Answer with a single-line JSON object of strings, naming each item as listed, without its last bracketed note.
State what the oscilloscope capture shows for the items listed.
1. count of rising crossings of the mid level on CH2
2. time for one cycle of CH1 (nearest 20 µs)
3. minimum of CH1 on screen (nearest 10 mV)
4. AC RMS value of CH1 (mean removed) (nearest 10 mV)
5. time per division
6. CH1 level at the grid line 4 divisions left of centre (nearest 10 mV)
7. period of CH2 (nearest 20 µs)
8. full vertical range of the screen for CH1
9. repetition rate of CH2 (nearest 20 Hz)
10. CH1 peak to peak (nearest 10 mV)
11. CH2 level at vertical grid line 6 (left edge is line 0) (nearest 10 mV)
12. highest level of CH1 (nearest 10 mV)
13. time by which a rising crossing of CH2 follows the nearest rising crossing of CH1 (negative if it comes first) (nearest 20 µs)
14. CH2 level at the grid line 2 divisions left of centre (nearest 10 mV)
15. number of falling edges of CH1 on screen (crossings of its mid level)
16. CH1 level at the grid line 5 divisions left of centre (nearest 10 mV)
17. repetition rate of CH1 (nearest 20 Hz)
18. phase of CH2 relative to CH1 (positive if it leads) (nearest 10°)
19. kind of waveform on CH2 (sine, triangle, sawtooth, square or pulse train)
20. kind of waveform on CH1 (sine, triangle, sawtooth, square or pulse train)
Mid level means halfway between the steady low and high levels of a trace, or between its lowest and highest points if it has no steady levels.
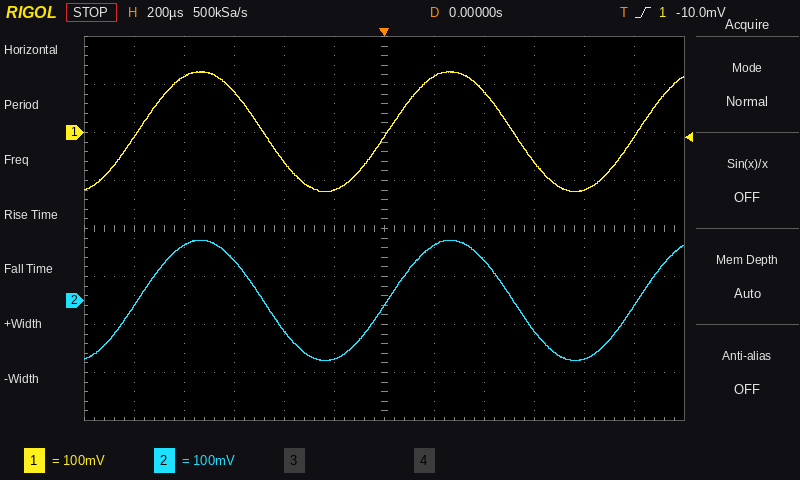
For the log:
{"count of rising crossings of the mid level on CH2": "3", "time for one cycle of CH1": "1.00 ms", "minimum of CH1 on screen": "-120 mV", "AC RMS value of CH1 (mean removed)": "90 mV", "time per division": "200 µs", "CH1 level at the grid line 4 divisions left of centre": "120 mV", "period of CH2": "1.00 ms", "full vertical range of the screen for CH1": "800 mV", "repetition rate of CH2": "1.00 kHz", "CH1 peak to peak": "250 mV", "CH2 level at vertical grid line 6 (left edge is line 0)": "-10 mV", "highest level of CH1": "130 mV", "time by which a rising crossing of CH2 follows the nearest rising crossing of CH1 (negative if it comes first)": "0 µs", "CH2 level at the grid line 2 divisions left of centre": "-60 mV", "number of falling edges of CH1 on screen": "2", "CH1 level at the grid line 5 divisions left of centre": "-10 mV", "repetition rate of CH1": "1.00 kHz", "phase of CH2 relative to CH1 (positive if it leads)": "0°", "kind of waveform on CH2": "sine", "kind of waveform on CH1": "sine"}
